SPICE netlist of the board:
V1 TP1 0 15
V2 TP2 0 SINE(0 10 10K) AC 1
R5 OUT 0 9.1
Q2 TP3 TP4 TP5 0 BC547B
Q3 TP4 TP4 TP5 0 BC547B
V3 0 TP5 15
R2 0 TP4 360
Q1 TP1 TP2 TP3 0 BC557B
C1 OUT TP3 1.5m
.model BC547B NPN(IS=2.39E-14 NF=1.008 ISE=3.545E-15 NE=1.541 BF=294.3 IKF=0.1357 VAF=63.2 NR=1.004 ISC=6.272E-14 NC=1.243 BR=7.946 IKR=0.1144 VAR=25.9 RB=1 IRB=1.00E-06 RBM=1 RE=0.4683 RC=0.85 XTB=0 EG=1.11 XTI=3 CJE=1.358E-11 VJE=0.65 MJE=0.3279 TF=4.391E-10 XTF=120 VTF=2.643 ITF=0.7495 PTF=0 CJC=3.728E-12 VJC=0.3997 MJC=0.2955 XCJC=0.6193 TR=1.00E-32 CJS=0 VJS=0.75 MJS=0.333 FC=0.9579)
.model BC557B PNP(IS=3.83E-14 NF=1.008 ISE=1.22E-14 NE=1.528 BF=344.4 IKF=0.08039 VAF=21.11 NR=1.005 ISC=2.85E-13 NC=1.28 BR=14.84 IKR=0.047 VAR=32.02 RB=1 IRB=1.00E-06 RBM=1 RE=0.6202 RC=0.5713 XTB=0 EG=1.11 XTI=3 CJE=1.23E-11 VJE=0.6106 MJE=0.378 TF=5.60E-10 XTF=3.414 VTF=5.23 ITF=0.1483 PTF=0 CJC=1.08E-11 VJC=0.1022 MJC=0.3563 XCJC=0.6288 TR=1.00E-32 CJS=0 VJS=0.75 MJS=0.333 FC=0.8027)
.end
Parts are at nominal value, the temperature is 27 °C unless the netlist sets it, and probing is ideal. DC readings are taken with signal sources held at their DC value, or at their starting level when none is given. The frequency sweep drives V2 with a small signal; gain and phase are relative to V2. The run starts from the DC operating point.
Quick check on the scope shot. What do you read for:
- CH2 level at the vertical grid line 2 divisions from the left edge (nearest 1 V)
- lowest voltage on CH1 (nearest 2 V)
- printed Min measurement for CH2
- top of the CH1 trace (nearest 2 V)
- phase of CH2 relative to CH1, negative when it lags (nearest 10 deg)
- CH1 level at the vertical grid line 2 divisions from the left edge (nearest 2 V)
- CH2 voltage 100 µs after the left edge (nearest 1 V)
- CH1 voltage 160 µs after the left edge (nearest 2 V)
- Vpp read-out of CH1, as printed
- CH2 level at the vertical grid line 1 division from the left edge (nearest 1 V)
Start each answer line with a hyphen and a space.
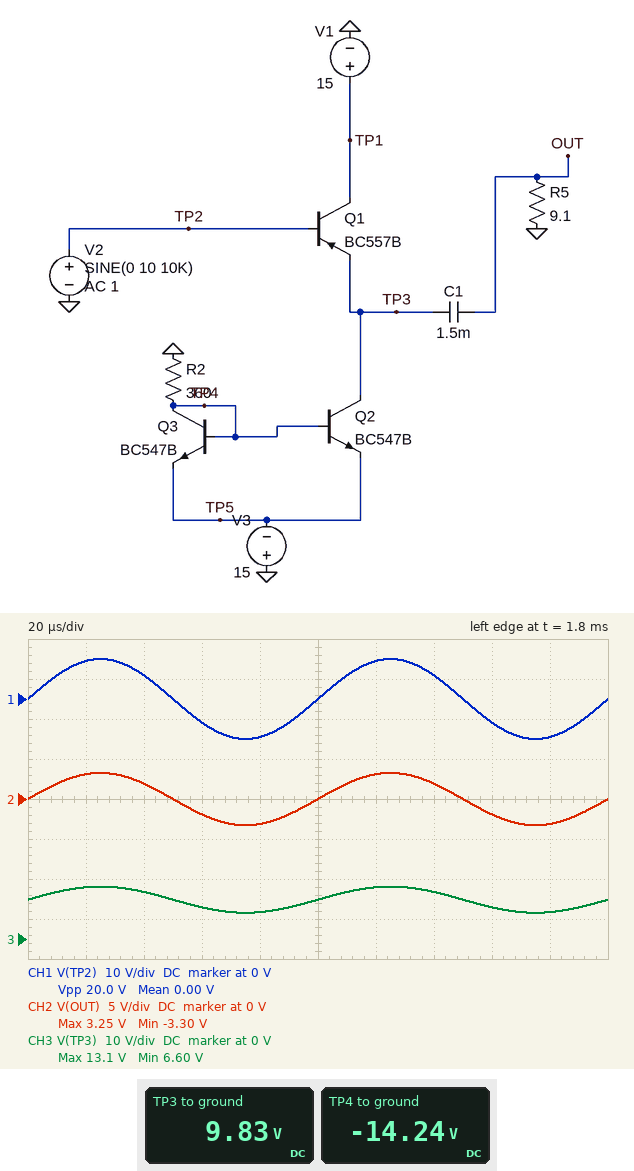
- 2 V
- -10 V
- -3.30 V
- 10 V
- 0 deg
- 6 V
- 0 V
- -6 V
- 20.0 V
- 3 V
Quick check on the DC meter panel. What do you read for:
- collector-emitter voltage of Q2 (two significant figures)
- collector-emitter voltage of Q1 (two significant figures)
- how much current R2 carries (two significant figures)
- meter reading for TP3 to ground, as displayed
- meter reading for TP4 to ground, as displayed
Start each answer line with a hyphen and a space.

- 25 V
- 5.2 V
- 40 mA
- 9.83 V
- -14.24 V
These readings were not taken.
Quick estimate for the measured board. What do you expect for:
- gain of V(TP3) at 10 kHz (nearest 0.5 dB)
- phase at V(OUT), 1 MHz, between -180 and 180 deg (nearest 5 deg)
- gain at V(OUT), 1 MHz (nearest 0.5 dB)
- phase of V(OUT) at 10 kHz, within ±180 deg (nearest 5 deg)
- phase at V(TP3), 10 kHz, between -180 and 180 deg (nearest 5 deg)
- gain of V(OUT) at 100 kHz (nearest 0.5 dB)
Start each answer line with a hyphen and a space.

- -9.5 dB
- 0 deg
- -9.5 dB
- 0 deg
- 0 deg
- -9.5 dB
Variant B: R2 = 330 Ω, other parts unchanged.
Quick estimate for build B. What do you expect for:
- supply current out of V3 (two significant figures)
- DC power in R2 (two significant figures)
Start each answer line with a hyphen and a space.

- 95 mA
- 610 mW
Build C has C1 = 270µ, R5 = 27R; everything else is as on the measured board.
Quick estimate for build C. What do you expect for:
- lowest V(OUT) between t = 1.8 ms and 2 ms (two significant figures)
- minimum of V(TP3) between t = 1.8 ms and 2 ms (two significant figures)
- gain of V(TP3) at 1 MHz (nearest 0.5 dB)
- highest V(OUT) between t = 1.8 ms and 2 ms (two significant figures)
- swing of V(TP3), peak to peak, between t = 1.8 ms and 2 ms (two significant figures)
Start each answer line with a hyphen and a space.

- -3.5 V
- 6.3 V
- -9.0 dB
- 3.5 V
- 7.0 V
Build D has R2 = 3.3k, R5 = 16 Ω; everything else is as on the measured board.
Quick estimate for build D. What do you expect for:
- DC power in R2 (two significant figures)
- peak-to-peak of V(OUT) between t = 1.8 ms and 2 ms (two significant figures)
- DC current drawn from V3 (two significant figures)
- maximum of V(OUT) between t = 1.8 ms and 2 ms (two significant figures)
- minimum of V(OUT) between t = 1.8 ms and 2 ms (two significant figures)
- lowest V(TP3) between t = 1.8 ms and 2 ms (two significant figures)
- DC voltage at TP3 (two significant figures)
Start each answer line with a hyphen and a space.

- 62 mW
- 6.8 V
- 10 mA
- 3.4 V
- -3.4 V
- 6.5 V
- 9.9 V
